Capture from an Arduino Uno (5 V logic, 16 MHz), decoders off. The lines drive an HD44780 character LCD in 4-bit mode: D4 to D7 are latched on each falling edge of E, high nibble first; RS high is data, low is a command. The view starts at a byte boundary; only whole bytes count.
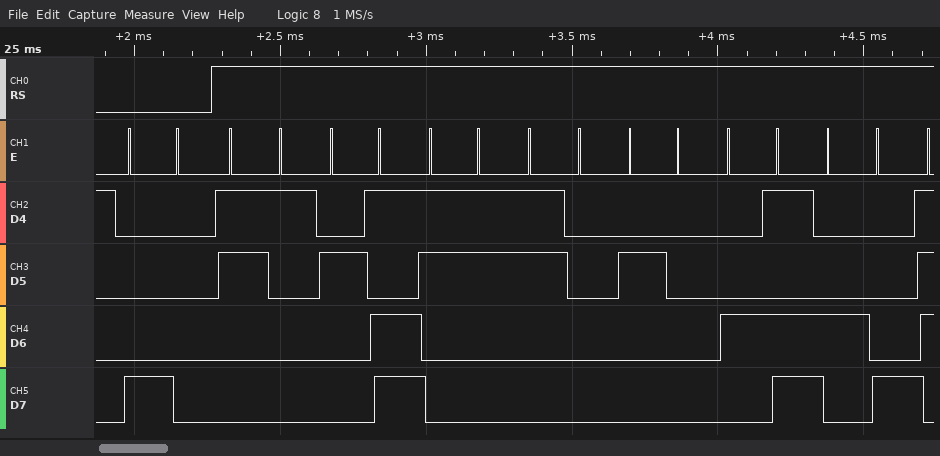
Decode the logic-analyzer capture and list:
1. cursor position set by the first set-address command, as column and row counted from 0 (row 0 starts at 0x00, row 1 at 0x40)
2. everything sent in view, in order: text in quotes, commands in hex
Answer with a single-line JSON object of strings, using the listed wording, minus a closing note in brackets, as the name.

{"cursor position set by the first set-address command, as column and row counted from 0": "column 0, row 0", "everything sent in view, in order: text in quotes, commands in hex": "0x80 \"1-30 MH\""}
